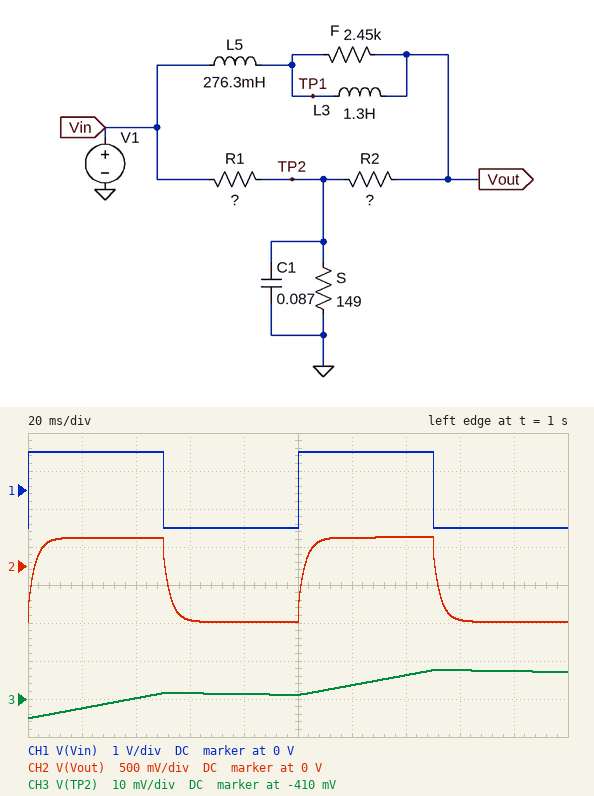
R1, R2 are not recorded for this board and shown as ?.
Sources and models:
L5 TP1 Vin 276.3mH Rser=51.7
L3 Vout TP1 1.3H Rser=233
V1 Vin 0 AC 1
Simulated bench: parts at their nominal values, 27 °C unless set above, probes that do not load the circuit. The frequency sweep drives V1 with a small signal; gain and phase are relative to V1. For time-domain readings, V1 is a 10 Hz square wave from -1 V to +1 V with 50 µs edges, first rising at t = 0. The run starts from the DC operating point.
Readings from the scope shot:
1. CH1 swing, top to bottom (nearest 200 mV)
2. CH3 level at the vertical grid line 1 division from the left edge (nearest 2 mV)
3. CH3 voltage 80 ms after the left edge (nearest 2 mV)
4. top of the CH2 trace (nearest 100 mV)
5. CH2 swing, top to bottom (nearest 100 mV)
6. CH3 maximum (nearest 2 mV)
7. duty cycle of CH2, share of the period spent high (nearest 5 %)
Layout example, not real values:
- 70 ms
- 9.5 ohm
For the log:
- 2.0 V
- -412 mV
- -408 mV
- 400 mV
- 1.1 V
- -402 mV
- 50 %
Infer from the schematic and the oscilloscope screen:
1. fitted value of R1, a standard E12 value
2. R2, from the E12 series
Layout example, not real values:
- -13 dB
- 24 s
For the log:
- 220 Ω
- 330 Ω
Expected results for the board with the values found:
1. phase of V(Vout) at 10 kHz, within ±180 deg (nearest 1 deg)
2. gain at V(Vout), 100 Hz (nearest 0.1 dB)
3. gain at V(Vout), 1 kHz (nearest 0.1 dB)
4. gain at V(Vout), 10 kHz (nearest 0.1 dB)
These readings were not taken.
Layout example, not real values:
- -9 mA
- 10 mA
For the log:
- -81 deg
- -10.6 dB
- -20.6 dB
- -34.6 dB
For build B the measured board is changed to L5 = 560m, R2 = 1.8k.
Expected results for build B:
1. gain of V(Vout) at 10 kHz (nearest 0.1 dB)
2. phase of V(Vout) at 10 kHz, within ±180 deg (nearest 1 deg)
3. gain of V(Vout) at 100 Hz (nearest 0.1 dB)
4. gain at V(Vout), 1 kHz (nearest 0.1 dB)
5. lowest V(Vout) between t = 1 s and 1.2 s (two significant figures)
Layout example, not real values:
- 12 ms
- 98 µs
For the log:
- -25.9 dB
- -83 deg
- -2.7 dB
- -10.2 dB
- -920 mV
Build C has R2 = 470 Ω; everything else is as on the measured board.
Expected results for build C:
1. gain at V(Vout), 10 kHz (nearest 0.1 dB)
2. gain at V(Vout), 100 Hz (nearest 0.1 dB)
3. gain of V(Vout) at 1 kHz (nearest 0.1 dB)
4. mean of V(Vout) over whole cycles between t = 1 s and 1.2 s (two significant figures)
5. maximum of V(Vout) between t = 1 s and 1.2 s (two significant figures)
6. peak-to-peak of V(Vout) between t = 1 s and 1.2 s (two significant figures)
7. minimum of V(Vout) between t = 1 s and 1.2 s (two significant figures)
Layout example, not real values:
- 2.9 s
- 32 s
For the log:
- -31.5 dB
- -8.3 dB
- -17.8 dB
- -140 mV
- 500 mV
- 1.3 V
- -790 mV
